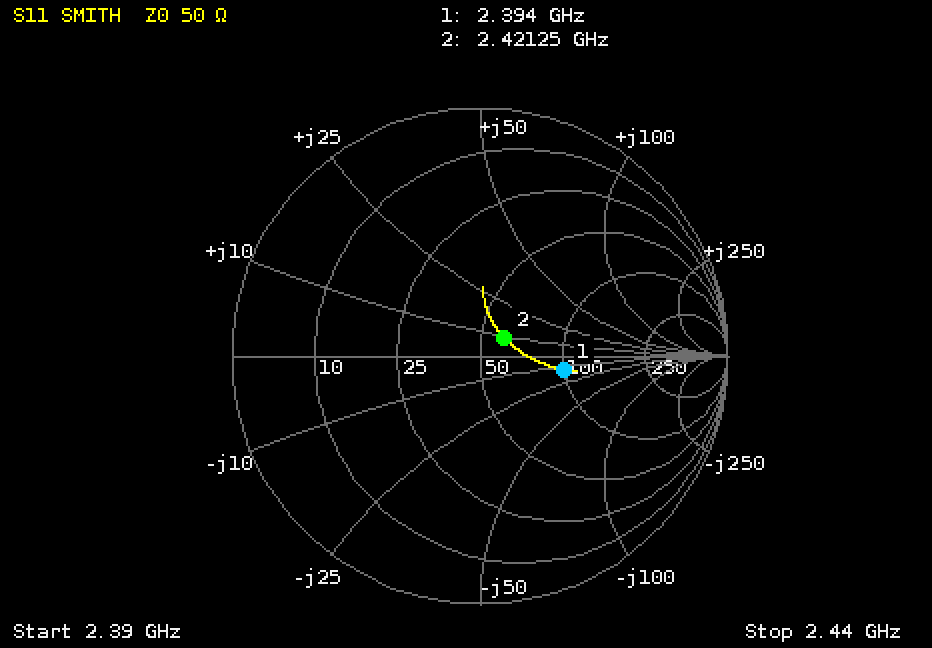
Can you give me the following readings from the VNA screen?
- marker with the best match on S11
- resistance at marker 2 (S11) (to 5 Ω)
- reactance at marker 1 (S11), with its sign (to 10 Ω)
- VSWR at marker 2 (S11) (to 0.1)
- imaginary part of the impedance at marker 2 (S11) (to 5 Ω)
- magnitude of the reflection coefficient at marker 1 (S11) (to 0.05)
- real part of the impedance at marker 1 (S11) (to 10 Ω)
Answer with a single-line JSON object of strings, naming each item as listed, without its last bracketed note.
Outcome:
{"marker with the best match on S11": "marker 2", "resistance at marker 2 (S11)": "60 Ω", "reactance at marker 1 (S11), with its sign": "-10 Ω", "VSWR at marker 2 (S11)": "1.3", "imaginary part of the impedance at marker 2 (S11)": "+10 Ω", "magnitude of the reflection coefficient at marker 1 (S11)": "0.35", "real part of the impedance at marker 1 (S11)": "100 Ω"}
